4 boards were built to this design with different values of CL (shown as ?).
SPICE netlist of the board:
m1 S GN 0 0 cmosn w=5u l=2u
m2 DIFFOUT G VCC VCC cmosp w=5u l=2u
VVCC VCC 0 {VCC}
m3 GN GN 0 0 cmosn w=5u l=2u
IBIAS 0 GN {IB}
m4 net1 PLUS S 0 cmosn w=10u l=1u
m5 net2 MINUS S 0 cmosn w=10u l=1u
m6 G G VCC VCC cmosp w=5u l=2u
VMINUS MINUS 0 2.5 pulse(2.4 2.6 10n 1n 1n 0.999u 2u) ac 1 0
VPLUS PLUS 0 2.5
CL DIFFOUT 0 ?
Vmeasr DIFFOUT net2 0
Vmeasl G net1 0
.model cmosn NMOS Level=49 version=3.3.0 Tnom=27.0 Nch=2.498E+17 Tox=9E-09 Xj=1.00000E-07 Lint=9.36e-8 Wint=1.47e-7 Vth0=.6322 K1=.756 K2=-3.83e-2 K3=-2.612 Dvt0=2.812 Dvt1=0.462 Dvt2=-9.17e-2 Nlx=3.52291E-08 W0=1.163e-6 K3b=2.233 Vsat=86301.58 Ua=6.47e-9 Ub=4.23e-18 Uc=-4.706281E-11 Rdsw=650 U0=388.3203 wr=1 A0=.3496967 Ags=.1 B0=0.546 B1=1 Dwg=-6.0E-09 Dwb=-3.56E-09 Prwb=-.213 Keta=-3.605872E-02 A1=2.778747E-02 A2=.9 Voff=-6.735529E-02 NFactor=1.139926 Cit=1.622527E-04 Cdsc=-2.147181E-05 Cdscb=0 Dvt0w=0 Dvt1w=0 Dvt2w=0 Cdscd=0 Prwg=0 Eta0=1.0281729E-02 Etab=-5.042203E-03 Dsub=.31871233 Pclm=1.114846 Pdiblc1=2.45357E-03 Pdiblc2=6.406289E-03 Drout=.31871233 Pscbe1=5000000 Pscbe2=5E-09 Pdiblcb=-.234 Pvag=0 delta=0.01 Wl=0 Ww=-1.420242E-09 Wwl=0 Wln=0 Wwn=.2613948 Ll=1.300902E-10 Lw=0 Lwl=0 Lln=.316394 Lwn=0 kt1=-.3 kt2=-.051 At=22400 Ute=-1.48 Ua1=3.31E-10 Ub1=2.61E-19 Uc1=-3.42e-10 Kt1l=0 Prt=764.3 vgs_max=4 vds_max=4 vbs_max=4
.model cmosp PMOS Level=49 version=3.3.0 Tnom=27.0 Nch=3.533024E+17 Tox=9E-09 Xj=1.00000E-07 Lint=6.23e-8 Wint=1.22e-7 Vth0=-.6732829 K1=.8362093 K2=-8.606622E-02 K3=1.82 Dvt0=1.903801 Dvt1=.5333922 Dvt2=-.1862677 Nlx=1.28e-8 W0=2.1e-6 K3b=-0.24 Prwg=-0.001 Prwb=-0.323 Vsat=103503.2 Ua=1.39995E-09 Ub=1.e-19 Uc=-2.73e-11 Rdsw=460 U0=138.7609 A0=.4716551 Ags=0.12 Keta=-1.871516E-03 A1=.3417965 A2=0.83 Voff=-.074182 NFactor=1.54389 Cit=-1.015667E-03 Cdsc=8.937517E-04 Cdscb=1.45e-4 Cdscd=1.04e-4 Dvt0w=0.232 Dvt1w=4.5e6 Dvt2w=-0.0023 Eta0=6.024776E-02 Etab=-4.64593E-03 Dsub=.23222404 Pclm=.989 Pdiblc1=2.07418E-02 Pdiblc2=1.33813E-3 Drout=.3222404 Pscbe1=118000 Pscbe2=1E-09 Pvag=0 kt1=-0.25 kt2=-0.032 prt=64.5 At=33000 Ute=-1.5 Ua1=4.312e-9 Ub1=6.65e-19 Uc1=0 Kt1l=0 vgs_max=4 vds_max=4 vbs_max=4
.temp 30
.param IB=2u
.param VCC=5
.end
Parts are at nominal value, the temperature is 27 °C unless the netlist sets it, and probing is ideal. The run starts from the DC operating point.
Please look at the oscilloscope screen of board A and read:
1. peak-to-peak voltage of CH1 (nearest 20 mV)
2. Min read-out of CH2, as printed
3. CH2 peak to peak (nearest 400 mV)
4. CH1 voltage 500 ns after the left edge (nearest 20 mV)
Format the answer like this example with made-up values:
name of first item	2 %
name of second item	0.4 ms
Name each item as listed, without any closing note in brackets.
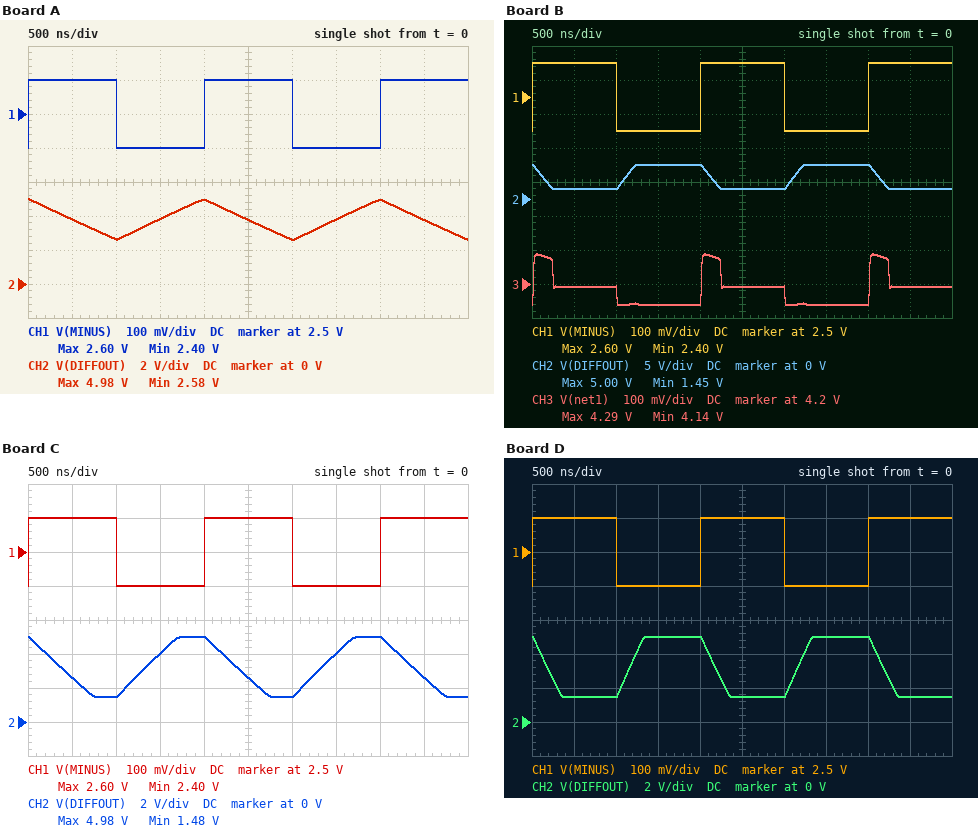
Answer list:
peak-to-peak voltage of CH1	200 mV
Min read-out of CH2, as printed	2.58 V
CH2 peak to peak	2.4 V
CH1 voltage 500 ns after the left edge	2.60 V
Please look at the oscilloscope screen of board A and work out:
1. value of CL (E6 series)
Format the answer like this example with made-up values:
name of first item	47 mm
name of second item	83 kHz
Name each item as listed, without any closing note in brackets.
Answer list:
value of CL	680 fF
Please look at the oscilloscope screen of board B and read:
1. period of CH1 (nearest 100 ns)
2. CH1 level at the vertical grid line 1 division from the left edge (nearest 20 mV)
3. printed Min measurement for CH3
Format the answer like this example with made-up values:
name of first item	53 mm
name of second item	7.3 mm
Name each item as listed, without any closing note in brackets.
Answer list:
period of CH1	2.0 µs
CH1 level at the vertical grid line 1 division from the left edge	2.60 V
printed Min measurement for CH3	4.14 V
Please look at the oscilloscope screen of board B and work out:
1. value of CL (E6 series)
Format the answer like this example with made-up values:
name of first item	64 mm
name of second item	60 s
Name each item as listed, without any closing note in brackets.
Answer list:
value of CL	100 fF
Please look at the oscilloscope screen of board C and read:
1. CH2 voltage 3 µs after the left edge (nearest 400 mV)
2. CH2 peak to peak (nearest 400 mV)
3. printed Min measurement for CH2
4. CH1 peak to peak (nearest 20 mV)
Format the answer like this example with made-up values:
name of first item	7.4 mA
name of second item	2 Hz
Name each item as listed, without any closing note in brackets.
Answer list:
CH2 voltage 3 µs after the left edge	1.6 V
CH2 peak to peak	3.6 V
printed Min measurement for CH2	1.48 V
CH1 peak to peak	200 mV
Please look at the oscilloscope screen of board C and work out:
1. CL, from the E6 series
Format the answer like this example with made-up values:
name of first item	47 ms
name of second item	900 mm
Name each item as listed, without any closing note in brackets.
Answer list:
CL, from the E6 series	330 fF
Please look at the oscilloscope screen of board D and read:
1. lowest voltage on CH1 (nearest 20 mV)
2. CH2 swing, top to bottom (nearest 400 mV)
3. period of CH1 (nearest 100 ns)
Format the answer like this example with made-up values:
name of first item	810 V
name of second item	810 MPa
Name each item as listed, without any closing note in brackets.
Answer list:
lowest voltage on CH1	2.40 V
CH2 swing, top to bottom	3.6 V
period of CH1	2.0 µs
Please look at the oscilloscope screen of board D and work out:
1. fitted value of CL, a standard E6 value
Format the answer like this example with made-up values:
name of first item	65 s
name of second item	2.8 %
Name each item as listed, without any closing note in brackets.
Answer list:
fitted value of CL, a standard E6 value	150 fF
